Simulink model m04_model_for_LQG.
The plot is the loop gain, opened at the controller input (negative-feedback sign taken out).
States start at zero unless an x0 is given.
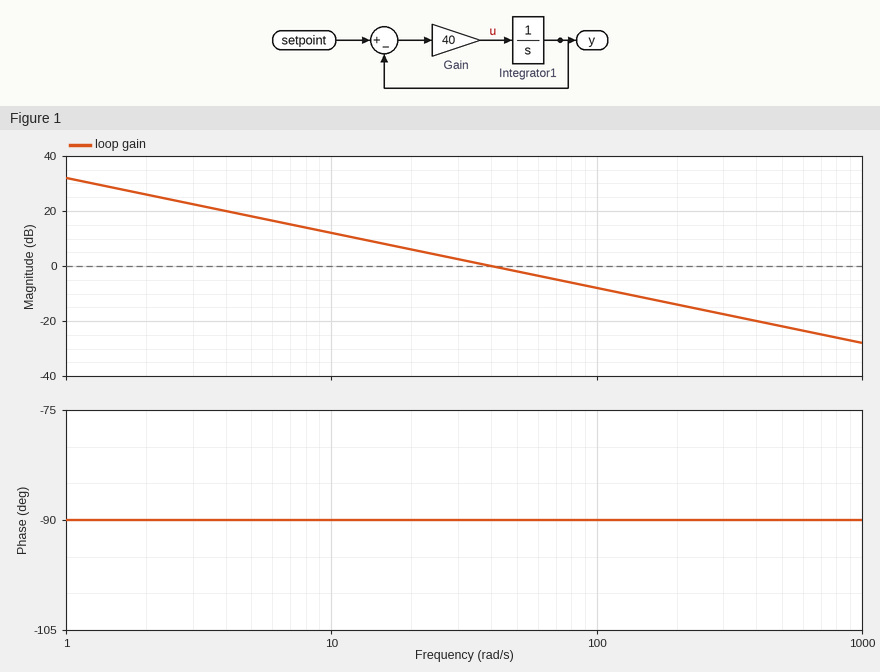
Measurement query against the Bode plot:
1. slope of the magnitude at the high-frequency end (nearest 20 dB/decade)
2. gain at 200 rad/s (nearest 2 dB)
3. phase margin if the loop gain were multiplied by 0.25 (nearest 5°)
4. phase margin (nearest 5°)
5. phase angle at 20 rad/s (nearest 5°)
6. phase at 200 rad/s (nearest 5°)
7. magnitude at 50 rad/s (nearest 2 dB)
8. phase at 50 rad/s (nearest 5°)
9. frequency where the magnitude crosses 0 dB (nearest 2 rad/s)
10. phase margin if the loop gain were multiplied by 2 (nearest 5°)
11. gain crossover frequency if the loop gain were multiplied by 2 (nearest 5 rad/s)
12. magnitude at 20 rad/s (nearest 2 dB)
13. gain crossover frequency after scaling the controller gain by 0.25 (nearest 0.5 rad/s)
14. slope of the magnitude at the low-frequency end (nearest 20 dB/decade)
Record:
-20 dB/decade
-14 dB
90°
90°
-90°
-90°
-2 dB
-90°
40 rad/s
90°
80 rad/s
6 dB
10.0 rad/s
-20 dB/decade
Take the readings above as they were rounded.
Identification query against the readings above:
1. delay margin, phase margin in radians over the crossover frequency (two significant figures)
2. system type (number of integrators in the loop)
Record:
0.039 s
1
